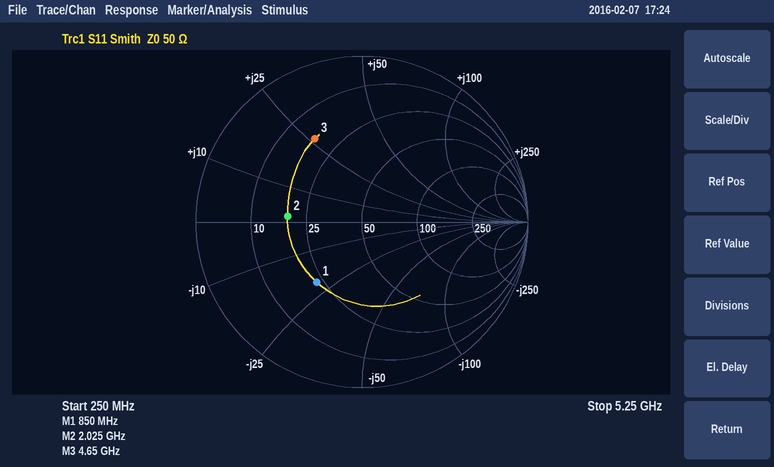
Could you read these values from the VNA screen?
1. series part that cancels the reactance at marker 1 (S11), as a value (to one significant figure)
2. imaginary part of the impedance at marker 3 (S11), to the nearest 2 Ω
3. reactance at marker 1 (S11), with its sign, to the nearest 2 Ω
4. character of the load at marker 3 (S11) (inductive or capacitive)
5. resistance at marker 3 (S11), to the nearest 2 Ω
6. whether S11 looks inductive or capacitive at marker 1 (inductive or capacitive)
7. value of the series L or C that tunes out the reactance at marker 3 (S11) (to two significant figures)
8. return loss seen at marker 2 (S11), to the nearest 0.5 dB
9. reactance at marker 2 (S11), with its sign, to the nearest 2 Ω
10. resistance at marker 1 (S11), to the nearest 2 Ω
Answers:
4 nH
+26 Ω
-20 Ω
inductive
18 Ω
capacitive
1.3 pF
7.0 dB
+2 Ω
22 Ω
